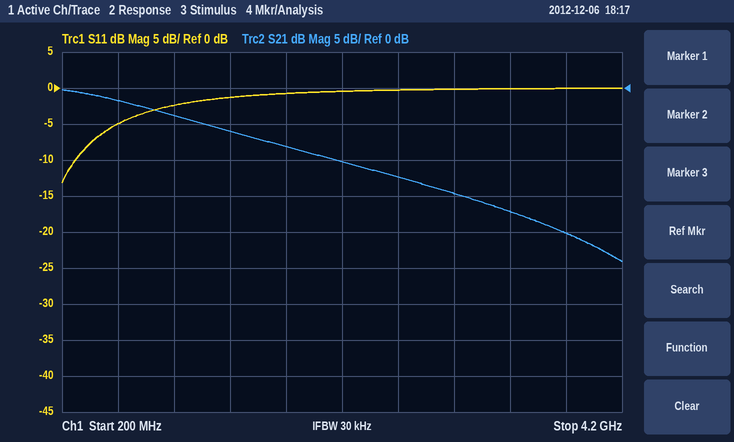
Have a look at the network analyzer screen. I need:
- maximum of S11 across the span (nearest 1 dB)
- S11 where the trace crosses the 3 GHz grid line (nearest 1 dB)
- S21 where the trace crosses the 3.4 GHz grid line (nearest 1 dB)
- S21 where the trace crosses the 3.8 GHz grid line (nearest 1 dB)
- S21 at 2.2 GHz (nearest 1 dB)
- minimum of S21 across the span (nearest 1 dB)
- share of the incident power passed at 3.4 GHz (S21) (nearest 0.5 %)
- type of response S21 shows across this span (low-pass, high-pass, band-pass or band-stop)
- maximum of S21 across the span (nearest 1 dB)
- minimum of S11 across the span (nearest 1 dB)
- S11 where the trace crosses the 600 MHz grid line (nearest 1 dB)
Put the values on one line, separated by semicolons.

0 dB; 0 dB; -17 dB; -20 dB; -10 dB; -24 dB; 2.0 %; low-pass; 0 dB; -13 dB; -5 dB
